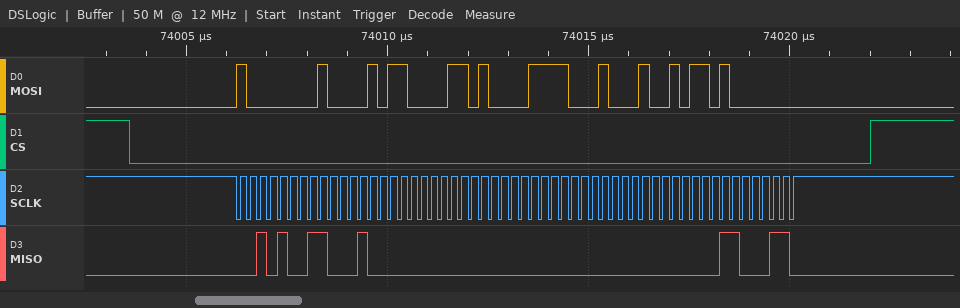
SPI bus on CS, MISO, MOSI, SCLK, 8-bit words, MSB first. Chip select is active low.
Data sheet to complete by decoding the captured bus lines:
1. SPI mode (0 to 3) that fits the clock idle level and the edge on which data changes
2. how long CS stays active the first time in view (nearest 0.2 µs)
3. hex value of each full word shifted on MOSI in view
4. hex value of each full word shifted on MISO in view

3
18.4 µs
80, 85, 86, 87, 88, 96, 80
29, 88, 00, 00, 00, 00, C6
